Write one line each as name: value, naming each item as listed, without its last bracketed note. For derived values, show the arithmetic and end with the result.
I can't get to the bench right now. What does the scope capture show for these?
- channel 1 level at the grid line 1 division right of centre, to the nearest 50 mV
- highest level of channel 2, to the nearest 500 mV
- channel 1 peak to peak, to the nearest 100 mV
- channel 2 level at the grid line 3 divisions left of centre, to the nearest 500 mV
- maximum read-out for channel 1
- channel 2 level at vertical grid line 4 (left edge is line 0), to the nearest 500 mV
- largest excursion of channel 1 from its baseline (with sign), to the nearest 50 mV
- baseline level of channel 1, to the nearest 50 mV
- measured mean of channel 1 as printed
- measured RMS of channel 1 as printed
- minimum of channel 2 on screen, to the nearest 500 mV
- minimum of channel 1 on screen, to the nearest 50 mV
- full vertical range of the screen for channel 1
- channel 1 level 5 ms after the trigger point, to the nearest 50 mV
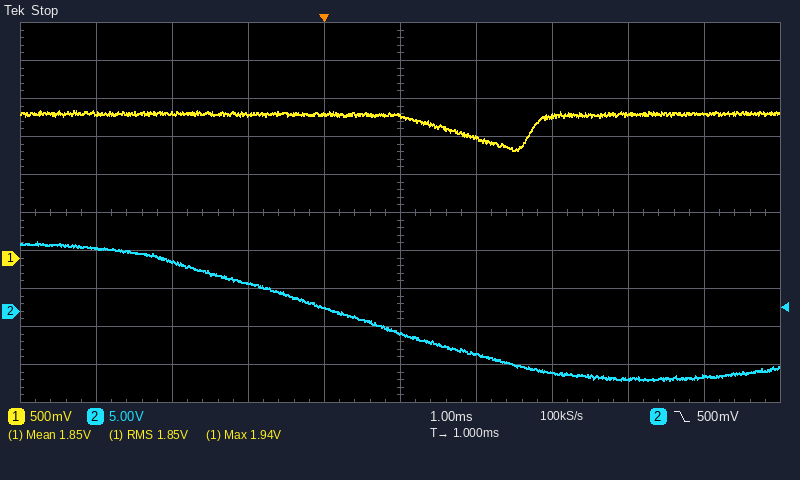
channel 1 level at the grid line 1 division right of centre, to the nearest 50 mV: 1.60 V
highest level of channel 2, to the nearest 500 mV: 9.0 V
channel 1 peak to peak, to the nearest 100 mV: 500 mV
channel 2 level at the grid line 3 divisions left of centre, to the nearest 500 mV: 6.5 V
maximum read-out for channel 1: 1.94 V
channel 2 level at vertical grid line 4 (left edge is line 0), to the nearest 500 mV: 500 mV
largest excursion of channel 1 from its baseline (with sign), to the nearest 50 mV: 1.40 V − (1.90 V) = -500 mV
baseline level of channel 1, to the nearest 50 mV: 1.90 V
measured mean of channel 1 as printed: 1.85 V
measured RMS of channel 1 as printed: 1.85 V
minimum of channel 2 on screen, to the nearest 500 mV: -9.0 V
minimum of channel 1 on screen, to the nearest 50 mV: 1.40 V
full vertical range of the screen for channel 1: 5 V
channel 1 level 5 ms after the trigger point, to the nearest 50 mV: 1.90 V
